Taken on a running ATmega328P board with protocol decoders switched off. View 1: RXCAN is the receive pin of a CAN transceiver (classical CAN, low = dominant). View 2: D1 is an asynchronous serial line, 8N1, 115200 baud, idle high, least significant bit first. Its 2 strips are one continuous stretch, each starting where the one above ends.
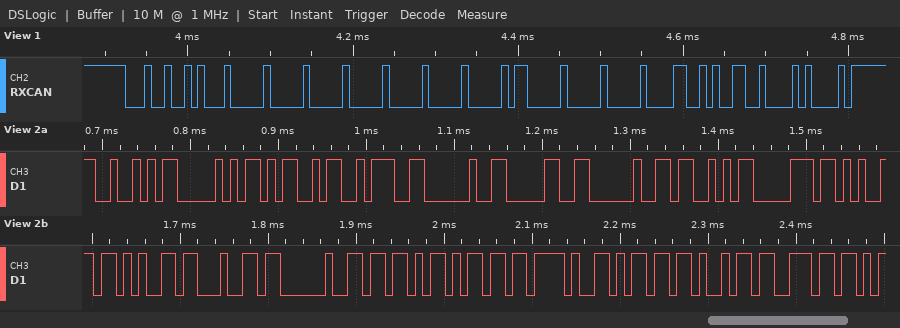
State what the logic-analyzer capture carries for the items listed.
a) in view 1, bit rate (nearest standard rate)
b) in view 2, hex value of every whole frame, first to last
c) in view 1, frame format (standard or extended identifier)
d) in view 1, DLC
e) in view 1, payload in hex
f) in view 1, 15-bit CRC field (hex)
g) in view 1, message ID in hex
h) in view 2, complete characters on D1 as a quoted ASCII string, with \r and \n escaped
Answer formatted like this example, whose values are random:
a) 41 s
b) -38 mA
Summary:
a) 125 kbit/s
b) 52 50 4D 3A 20 30 20 53 70 65 65 64 20 5B 6D 2F 6D 69 6E
c) standard
d) 8
e) 00 00 00 00 60 00 03 29
f) 0x4850
g) 0x125
h) "RPM: 0 Speed [m/min"
